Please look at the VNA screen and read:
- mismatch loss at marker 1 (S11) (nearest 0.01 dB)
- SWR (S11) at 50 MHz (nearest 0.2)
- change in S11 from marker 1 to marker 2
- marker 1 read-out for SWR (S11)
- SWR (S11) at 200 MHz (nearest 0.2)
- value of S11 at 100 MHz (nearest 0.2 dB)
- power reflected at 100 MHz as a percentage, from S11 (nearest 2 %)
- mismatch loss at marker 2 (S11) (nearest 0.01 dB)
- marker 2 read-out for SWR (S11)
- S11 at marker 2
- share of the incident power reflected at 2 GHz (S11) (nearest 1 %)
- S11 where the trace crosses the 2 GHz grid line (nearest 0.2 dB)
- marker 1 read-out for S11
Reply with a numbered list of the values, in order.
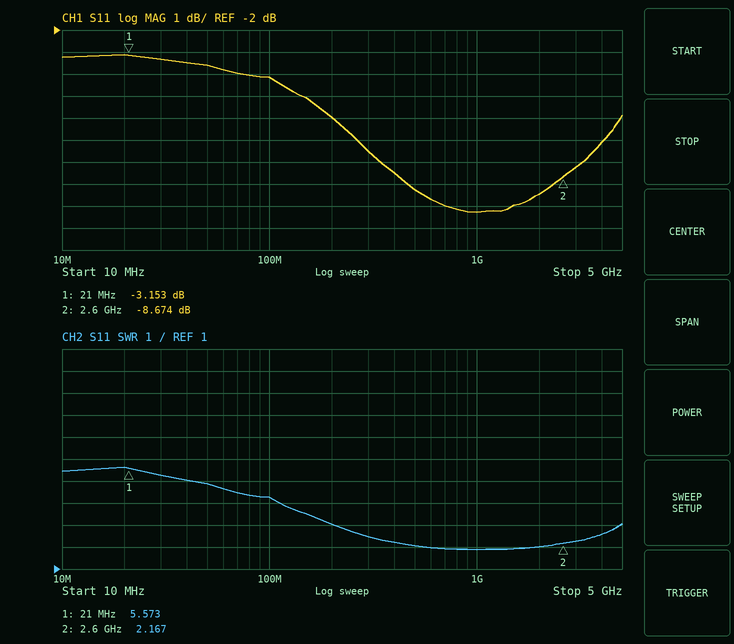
1. 2.87 dB
2. 4.8
3. -5.521 dB
4. 5.573
5. 3.0
6. -4.2 dB
7. 38 %
8. 0.63 dB
9. 2.167
10. -8.674 dB
11. 11 %
12. -9.4 dB
13. -3.153 dB
